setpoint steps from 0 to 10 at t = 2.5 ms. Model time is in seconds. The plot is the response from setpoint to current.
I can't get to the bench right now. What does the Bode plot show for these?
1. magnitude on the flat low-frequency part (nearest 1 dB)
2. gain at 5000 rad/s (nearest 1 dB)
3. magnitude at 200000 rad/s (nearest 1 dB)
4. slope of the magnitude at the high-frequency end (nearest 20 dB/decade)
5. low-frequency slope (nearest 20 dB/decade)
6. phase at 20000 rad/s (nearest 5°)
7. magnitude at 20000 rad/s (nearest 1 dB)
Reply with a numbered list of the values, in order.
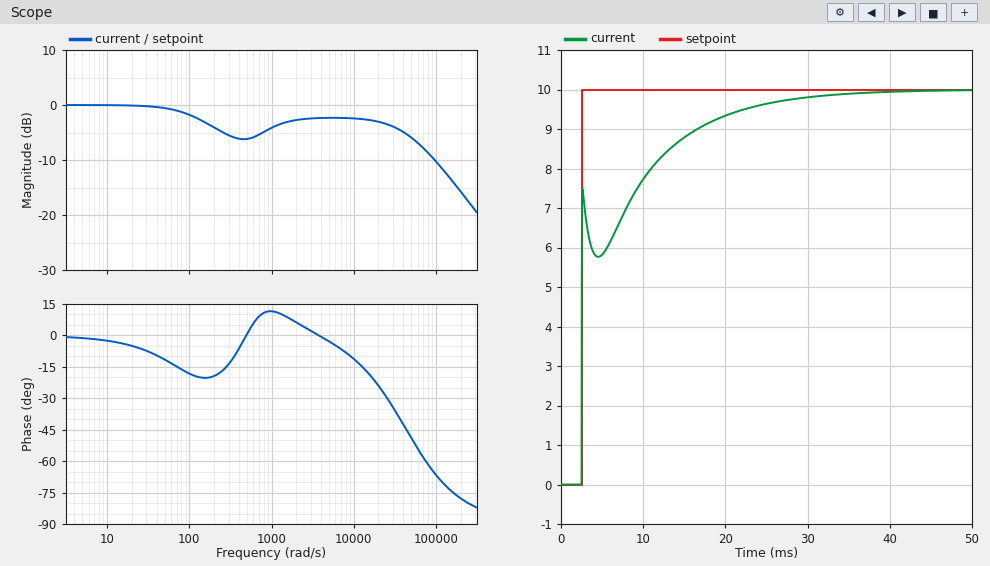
1. 0 dB
2. -2 dB
3. -16 dB
4. -20 dB/decade
5. 0 dB/decade
6. -25°
7. -3 dB
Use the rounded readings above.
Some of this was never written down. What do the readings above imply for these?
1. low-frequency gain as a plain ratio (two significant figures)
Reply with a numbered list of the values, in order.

1. 1.0
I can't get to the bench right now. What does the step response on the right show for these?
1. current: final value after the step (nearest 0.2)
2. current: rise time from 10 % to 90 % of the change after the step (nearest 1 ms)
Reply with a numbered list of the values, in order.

1. 10.0
2. 14 ms
